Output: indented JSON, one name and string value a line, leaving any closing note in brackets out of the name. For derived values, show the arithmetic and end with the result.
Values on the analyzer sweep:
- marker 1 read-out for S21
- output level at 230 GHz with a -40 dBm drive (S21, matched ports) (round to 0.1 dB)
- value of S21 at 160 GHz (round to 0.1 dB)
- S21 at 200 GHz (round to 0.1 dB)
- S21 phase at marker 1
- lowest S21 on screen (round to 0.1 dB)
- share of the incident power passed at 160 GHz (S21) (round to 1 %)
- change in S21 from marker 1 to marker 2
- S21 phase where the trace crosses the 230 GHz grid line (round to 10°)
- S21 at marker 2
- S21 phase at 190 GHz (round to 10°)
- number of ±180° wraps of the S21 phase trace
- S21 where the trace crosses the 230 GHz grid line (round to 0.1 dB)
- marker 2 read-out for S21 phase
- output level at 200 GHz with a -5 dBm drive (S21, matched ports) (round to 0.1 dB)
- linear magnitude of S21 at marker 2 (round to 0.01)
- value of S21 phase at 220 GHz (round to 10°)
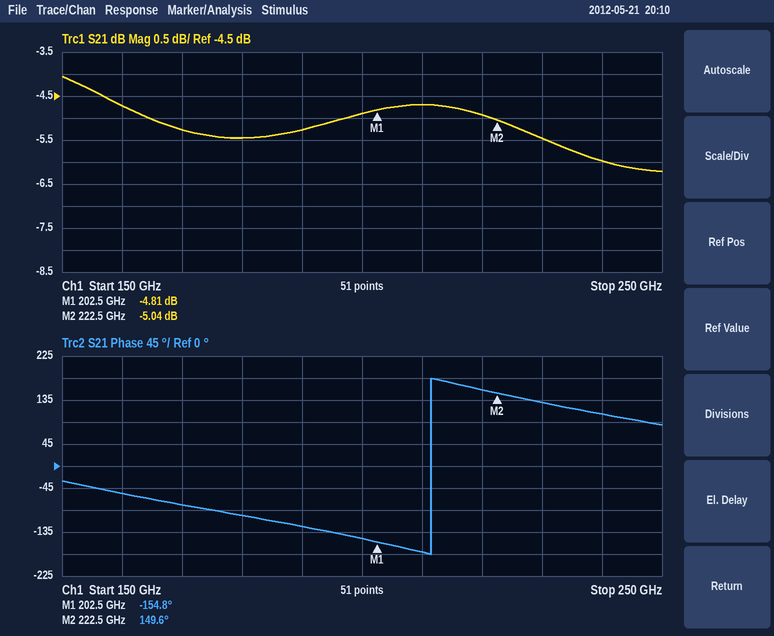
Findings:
{
  "marker 1 read-out for S21": "-4.81 dB",
  "output level at 230 GHz with a -40 dBm drive (S21, matched ports)": "-40 dBm + (-5.5 dB) = -45.5 dBm",
  "value of S21 at 160 GHz": "-4.7 dB",
  "S21 at 200 GHz": "-4.9 dB",
  "S21 phase at marker 1": "-154.8°",
  "lowest S21 on screen": "-6.2 dB",
  "share of the incident power passed at 160 GHz (S21)": "10^(-4.7/10) ≈ 34 %",
  "change in S21 from marker 1 to marker 2": "-5.04 − (-4.81) = -0.23 dB",
  "S21 phase where the trace crosses the 230 GHz grid line": "130°",
  "S21 at marker 2": "-5.04 dB",
  "S21 phase at 190 GHz": "-120°",
  "number of ±180° wraps of the S21 phase trace": "1",
  "S21 where the trace crosses the 230 GHz grid line": "-5.5 dB",
  "marker 2 read-out for S21 phase": "149.6°",
  "output level at 200 GHz with a -5 dBm drive (S21, matched ports)": "-5 dBm + (-4.9 dB) = -9.9 dBm",
  "linear magnitude of S21 at marker 2": "10^(-5.04/20) ≈ 0.56",
  "value of S21 phase at 220 GHz": "160°"
}
